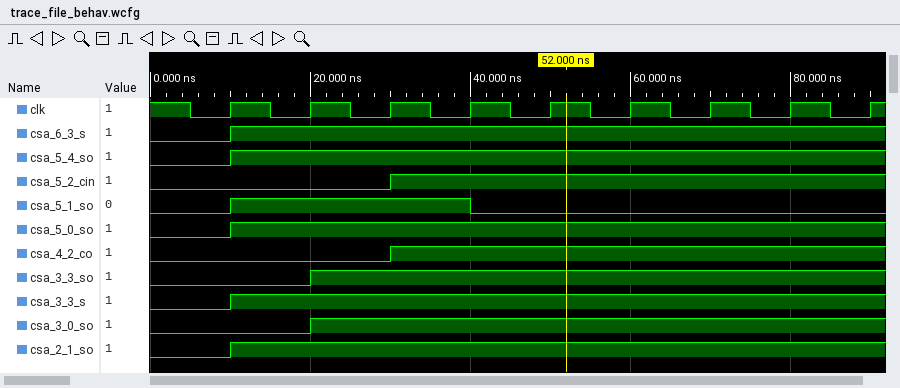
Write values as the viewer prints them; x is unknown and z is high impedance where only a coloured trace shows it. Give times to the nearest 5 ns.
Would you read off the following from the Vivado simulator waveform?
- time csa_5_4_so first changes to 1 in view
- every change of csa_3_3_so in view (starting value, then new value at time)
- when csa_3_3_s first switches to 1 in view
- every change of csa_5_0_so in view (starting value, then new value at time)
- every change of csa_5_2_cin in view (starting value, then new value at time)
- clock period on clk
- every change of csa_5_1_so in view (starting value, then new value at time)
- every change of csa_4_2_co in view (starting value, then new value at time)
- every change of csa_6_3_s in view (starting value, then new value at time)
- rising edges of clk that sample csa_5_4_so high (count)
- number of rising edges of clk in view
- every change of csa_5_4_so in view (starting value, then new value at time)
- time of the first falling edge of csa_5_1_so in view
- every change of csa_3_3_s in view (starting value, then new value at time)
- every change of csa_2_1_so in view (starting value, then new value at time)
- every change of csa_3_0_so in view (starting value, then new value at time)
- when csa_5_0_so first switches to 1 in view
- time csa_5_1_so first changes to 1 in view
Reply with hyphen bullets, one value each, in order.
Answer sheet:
- 10 ns
- 0, 1 at 20 ns
- 10 ns
- 0, 1 at 10 ns
- 0, 1 at 30 ns
- 10 ns
- 0, 1 at 10 ns, 0 at 40 ns
- 0, 1 at 30 ns
- 0, 1 at 10 ns
- 8
- 9
- 0, 1 at 10 ns
- 40 ns
- 0, 1 at 10 ns
- 0, 1 at 10 ns
- 0, 1 at 20 ns
- 10 ns
- 10 ns
